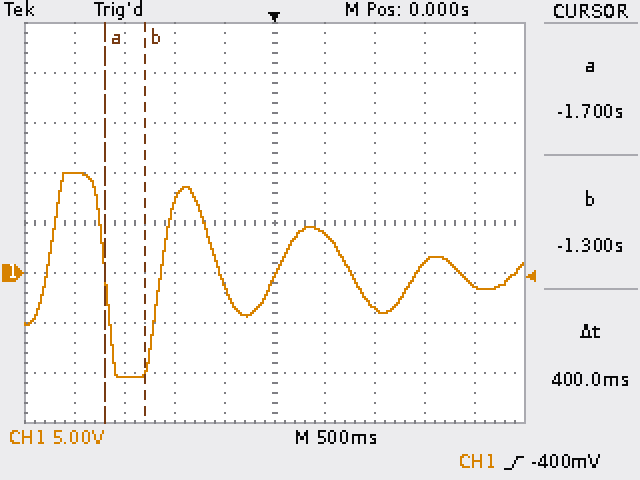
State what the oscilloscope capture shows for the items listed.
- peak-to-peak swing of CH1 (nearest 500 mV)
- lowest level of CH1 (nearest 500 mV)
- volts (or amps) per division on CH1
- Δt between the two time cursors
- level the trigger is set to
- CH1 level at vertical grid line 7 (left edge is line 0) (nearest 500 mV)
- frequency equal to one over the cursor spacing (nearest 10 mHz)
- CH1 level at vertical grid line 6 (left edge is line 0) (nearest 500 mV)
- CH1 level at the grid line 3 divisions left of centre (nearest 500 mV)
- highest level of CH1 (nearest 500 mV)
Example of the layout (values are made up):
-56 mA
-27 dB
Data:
20.5 V
-10.5 V
5 V
400 ms
-400 mV
-3.5 V
2.50 Hz
4.0 V
-10.5 V
10.0 V
